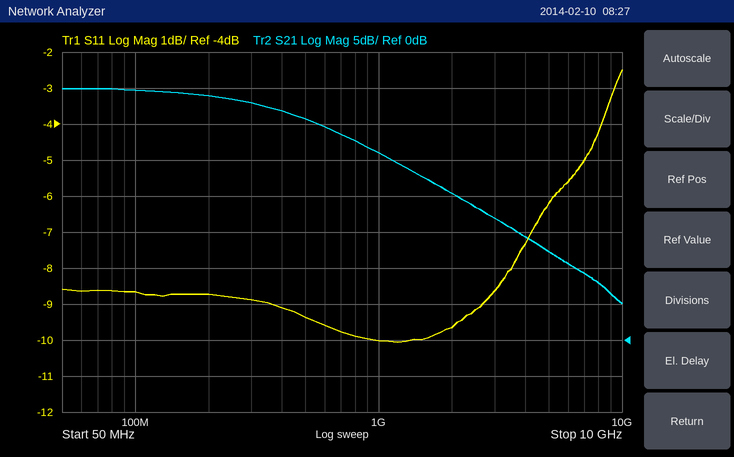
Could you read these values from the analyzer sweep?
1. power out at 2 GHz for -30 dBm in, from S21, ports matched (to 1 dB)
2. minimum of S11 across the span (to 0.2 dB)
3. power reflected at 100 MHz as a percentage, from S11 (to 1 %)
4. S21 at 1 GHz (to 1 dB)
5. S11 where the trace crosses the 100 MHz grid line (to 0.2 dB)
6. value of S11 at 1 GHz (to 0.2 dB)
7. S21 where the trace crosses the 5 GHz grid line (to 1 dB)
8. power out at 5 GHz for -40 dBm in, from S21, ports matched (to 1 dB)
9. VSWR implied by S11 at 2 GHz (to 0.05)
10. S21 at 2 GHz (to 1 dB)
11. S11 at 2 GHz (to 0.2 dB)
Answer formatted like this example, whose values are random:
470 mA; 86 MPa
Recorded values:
-10 dBm; -10.0 dB; 14 %; 26 dB; -8.6 dB; -10.0 dB; 12 dB; -28 dBm; 2.00; 20 dB; -9.6 dB
